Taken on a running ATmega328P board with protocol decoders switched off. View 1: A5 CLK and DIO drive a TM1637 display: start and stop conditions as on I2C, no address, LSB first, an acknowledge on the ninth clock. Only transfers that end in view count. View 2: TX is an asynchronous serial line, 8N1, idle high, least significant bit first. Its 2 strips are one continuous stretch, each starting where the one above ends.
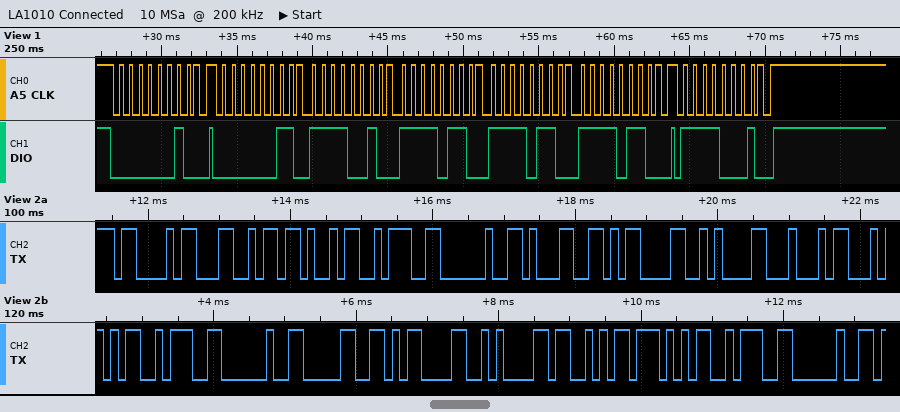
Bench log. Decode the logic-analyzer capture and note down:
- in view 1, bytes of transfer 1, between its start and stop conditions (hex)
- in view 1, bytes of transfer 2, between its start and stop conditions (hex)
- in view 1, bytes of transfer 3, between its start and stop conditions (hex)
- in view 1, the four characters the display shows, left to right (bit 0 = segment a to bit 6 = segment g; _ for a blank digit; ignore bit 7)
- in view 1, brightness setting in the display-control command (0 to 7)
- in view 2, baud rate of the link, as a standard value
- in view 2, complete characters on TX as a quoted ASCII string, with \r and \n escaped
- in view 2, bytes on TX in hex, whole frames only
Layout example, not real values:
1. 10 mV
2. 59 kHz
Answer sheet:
1. 40
2. C0 4F 6F 6F 6F
3. 8F
4. 3999
5. 7
6. 9600 baud
7. "CLK: 1\r\nDT: 0\r\nSW: "
8. 0x43 0x4C 0x4B 0x3A 0x20 0x31 0x0D 0x0A 0x44 0x54 0x3A 0x20 0x30 0x0D 0x0A 0x53 0x57 0x3A 0x20
